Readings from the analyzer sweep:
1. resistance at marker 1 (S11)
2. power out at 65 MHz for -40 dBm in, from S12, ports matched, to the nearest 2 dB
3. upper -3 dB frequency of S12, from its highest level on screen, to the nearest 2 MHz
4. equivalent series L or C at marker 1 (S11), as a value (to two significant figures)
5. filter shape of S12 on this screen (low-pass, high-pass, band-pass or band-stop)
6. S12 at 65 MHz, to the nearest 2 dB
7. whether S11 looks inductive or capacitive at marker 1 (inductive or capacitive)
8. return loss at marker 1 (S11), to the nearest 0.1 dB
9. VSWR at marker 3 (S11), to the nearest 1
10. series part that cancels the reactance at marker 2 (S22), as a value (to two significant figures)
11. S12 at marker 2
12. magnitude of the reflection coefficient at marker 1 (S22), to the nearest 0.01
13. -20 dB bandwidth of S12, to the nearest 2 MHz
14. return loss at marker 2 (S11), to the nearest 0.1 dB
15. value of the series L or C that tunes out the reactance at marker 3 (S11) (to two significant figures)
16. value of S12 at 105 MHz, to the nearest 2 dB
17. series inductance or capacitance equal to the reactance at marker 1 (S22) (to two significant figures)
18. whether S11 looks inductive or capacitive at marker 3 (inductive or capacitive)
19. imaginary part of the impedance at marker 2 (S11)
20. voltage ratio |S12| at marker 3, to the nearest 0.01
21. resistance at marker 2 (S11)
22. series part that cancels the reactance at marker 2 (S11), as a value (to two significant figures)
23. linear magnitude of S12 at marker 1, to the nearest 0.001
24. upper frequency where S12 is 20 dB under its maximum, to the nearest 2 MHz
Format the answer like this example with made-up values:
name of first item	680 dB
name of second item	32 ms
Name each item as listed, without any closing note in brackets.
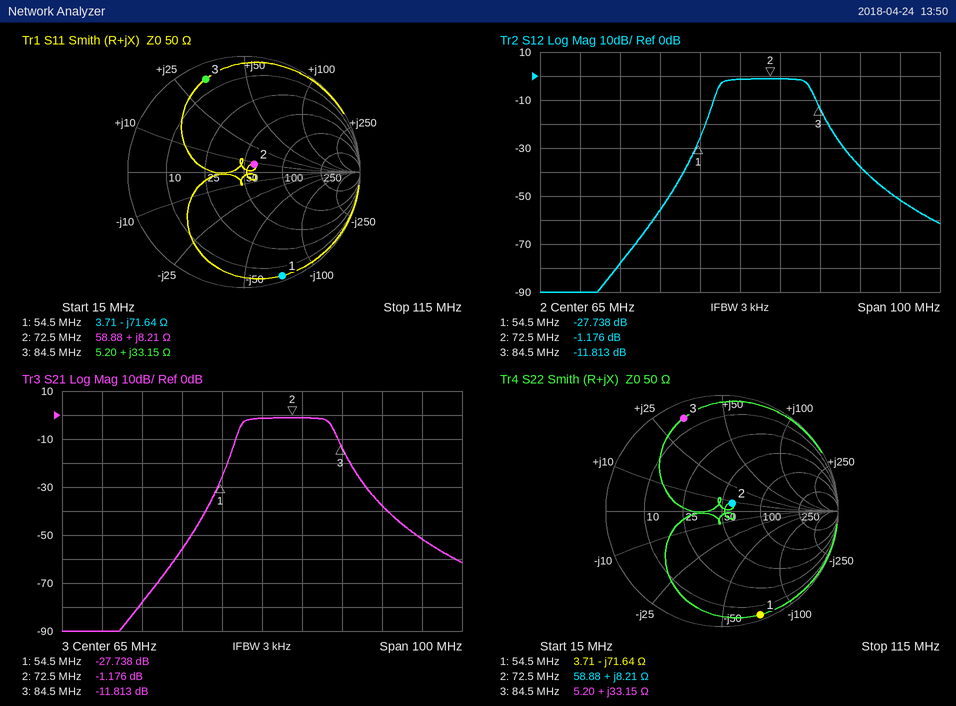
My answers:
resistance at marker 1	3.71 Ω
power out at 65 MHz for -40 dBm in, from S12, ports matched, to the nearest 2 dB	-42 dBm
upper -3 dB frequency of S12, from its highest level on screen, to the nearest 2 MHz	82 MHz
equivalent series L or C at marker 1 (S11), as a value	41 pF
filter shape of S12 on this screen	band-pass
S12 at 65 MHz, to the nearest 2 dB	-2 dB
whether S11 looks inductive or capacitive at marker 1	capacitive
return loss at marker 1 (S11), to the nearest 0.1 dB	0.4 dB
VSWR at marker 3 (S11), to the nearest 1	14
series part that cancels the reactance at marker 2 (S22), as a value	270 pF
S12 at marker 2	-1.176 dB
magnitude of the reflection coefficient at marker 1 (S22), to the nearest 0.01	0.95
-20 dB bandwidth of S12, to the nearest 2 MHz	32 MHz
return loss at marker 2 (S11), to the nearest 0.1 dB	19.1 dB
value of the series L or C that tunes out the reactance at marker 3 (S11)	57 pF
value of S12 at 105 MHz, to the nearest 2 dB	-52 dB
series inductance or capacitance equal to the reactance at marker 1 (S22)	41 pF
whether S11 looks inductive or capacitive at marker 3	inductive
imaginary part of the impedance at marker 2	+8.21 Ω
voltage ratio |S12| at marker 3, to the nearest 0.01	0.26
resistance at marker 2	58.88 Ω
series part that cancels the reactance at marker 2 (S11), as a value	270 pF
linear magnitude of S12 at marker 1, to the nearest 0.001	0.041
upper frequency where S12 is 20 dB under its maximum, to the nearest 2 MHz	88 MHz
